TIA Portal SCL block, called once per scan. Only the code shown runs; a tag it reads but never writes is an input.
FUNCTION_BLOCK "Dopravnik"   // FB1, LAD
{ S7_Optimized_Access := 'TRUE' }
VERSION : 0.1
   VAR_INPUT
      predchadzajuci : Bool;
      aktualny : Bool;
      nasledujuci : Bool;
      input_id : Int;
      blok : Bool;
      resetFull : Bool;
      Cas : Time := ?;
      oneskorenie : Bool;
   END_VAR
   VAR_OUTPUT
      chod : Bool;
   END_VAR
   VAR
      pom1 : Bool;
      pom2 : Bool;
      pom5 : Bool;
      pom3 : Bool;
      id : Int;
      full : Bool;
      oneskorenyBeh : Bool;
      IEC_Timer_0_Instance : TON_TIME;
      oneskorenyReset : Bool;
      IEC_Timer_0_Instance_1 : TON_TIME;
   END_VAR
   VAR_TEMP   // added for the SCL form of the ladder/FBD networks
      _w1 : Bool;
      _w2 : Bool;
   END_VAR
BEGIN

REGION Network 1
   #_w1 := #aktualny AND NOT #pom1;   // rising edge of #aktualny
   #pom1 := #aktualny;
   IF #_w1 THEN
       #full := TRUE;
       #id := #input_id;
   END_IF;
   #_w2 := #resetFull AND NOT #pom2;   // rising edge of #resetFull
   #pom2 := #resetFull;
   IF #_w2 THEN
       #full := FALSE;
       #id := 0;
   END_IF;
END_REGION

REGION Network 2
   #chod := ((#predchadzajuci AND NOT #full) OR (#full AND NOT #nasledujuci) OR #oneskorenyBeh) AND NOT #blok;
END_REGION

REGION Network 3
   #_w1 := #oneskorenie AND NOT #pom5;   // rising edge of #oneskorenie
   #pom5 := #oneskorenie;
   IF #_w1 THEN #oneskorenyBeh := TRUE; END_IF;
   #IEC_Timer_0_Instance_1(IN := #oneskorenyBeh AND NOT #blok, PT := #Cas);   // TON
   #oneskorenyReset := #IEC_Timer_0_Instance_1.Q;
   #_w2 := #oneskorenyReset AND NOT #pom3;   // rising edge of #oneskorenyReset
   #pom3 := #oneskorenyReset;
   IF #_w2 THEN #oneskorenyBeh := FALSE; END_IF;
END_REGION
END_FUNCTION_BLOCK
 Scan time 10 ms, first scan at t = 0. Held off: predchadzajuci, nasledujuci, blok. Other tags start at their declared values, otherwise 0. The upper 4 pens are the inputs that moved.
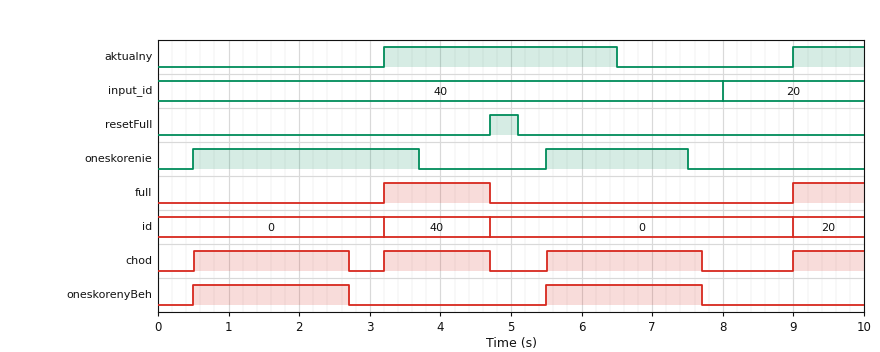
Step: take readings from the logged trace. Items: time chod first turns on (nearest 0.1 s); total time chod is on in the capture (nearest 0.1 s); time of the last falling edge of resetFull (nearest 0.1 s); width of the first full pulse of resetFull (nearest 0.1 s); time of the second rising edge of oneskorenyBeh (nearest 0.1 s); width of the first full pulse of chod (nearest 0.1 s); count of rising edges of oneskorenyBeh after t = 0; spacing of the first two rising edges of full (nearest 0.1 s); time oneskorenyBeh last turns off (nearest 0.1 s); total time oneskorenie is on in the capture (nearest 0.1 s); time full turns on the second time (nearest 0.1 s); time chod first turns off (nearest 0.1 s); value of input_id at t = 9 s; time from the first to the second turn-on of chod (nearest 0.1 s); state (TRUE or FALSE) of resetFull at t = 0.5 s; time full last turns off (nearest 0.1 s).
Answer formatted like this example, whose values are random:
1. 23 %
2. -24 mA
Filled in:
1. 0.5 s
2. 6.9 s
3. 5.1 s
4. 0.4 s
5. 5.5 s
6. 2.2 s
7. 2
8. 5.8 s
9. 7.7 s
10. 5.2 s
11. 9.0 s
12. 2.7 s
13. 20
14. 2.7 s
15. FALSE
16. 4.7 s
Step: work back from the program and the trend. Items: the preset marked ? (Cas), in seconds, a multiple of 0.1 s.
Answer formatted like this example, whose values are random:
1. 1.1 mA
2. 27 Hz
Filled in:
1. 2.2 s
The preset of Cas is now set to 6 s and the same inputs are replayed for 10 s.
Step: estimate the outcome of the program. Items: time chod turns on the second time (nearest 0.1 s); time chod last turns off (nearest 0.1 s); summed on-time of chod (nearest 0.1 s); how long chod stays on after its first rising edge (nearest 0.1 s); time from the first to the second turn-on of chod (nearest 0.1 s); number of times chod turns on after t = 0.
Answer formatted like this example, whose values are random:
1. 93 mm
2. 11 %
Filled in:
1. 9.0 s
2. 6.5 s
3. 7.0 s
4. 6.0 s
5. 8.5 s
6. 2
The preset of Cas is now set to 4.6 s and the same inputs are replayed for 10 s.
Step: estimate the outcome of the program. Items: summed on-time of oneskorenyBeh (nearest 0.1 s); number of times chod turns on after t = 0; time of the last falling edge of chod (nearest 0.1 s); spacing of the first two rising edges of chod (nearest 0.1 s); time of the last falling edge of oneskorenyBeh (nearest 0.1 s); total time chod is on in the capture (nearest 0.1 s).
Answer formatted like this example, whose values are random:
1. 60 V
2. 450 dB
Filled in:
1. 9.1 s
2. 2
3. 5.1 s
4. 5.0 s
5. 5.1 s
6. 9.1 s
